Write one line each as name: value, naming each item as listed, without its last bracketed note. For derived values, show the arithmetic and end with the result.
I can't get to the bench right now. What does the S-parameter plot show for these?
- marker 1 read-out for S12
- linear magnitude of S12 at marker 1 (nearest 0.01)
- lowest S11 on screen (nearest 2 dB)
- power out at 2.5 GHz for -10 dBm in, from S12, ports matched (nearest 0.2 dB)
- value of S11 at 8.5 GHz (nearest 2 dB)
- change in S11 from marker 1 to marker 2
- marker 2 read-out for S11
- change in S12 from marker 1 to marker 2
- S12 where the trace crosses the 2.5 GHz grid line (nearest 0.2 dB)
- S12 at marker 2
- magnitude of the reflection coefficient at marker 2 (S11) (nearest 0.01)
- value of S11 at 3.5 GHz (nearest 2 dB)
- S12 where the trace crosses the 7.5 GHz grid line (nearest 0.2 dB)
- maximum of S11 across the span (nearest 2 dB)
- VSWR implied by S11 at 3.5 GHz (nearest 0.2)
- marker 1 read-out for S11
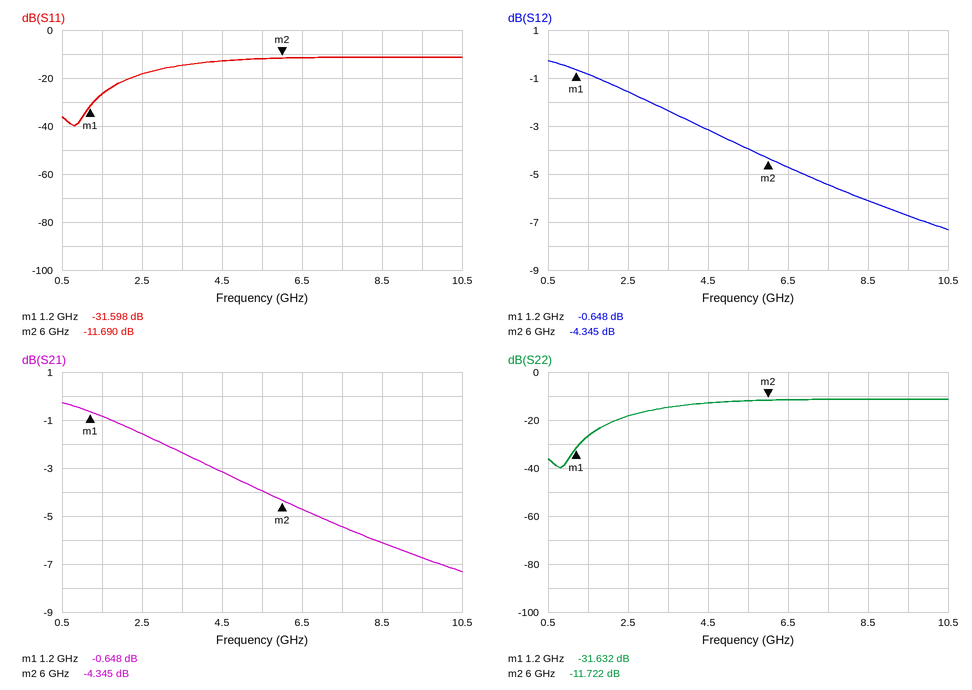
marker 1 read-out for S12: -0.648 dB
linear magnitude of S12 at marker 1: 10^(-0.648/20) ≈ 0.93
lowest S11 on screen: -40 dB
power out at 2.5 GHz for -10 dBm in, from S12, ports matched: -10 dBm + (-1.6 dB) = -11.6 dBm
value of S11 at 8.5 GHz: -12 dB
change in S11 from marker 1 to marker 2: -11.69 − (-31.598) = 19.908 dB
marker 2 read-out for S11: -11.690 dB
change in S12 from marker 1 to marker 2: -4.345 − (-0.648) = -3.697 dB
S12 where the trace crosses the 2.5 GHz grid line: -1.6 dB
S12 at marker 2: -4.345 dB
magnitude of the reflection coefficient at marker 2 (S11): 10^(-11.69/20) ≈ 0.26
value of S11 at 3.5 GHz: -14 dB
S12 where the trace crosses the 7.5 GHz grid line: -5.4 dB
maximum of S11 across the span: -12 dB
VSWR implied by S11 at 3.5 GHz: |Γ| = 10^(-14/20) = 0.1995; VSWR = (1 + 0.1995)/(1 − 0.1995) ≈ 1.50, so 1.4 to the nearest 0.2
marker 1 read-out for S11: -31.598 dB
